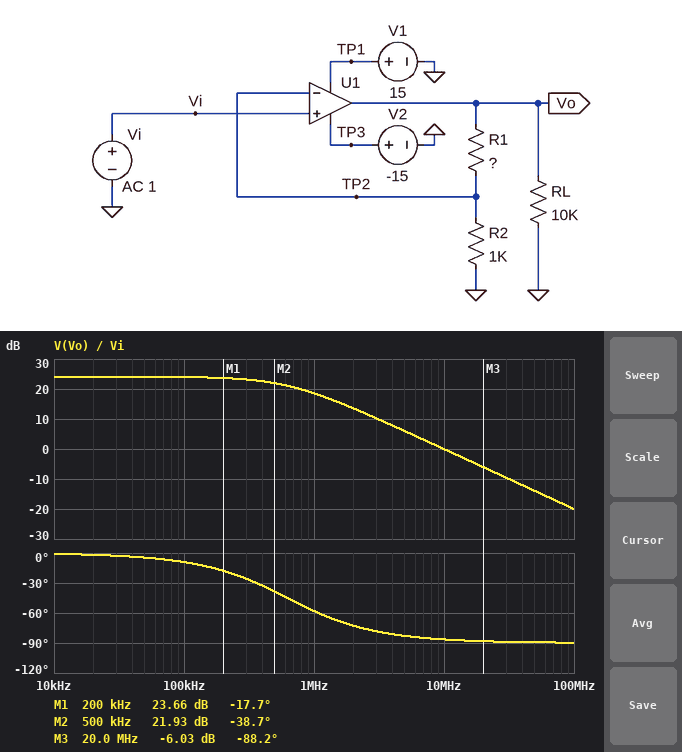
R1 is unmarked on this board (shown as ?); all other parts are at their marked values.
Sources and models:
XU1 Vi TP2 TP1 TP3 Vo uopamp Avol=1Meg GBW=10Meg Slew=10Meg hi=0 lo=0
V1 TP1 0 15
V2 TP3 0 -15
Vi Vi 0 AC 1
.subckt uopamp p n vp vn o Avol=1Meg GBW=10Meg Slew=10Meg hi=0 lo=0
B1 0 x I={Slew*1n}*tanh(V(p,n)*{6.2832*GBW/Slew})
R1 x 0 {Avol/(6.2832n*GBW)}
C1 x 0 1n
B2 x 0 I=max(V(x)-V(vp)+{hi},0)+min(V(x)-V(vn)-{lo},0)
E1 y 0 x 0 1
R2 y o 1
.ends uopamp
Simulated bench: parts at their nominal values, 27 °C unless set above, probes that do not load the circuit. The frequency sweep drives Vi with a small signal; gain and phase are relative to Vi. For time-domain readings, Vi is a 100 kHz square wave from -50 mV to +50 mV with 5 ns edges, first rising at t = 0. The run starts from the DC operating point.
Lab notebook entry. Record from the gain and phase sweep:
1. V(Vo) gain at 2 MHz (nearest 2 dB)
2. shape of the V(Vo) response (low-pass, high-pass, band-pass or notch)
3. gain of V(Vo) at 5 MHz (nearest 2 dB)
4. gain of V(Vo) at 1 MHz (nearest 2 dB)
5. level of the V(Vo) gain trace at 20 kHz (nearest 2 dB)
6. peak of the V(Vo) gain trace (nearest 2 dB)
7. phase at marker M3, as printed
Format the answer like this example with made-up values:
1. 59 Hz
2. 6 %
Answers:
1. 14 dB
2. low-pass
3. 6 dB
4. 18 dB
5. 24 dB
6. 24 dB
7. -88.2 deg
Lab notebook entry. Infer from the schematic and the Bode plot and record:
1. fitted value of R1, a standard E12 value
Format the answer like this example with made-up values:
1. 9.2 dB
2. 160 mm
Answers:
1. 15 kΩ
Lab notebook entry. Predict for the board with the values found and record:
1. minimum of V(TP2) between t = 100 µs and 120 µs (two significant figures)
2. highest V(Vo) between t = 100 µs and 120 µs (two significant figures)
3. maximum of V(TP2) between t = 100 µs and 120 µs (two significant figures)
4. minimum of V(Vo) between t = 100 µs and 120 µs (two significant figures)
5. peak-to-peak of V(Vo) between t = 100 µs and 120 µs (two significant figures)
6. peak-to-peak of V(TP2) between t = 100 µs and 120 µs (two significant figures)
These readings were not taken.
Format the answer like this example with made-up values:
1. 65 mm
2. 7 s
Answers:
1. -50 mV
2. 800 mV
3. 50 mV
4. -800 mV
5. 1.6 V
6. 100 mV
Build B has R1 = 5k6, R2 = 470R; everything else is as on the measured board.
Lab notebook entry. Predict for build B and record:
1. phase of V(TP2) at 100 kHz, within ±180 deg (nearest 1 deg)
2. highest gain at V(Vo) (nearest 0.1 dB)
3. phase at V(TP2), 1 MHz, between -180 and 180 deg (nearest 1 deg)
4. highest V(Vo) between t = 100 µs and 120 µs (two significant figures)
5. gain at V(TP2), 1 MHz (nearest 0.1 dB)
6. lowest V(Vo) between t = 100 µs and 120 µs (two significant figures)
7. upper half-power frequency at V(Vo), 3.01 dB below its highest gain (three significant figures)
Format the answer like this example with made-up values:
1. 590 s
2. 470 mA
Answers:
1. -7 deg
2. 22.2 dB
3. -52 deg
4. 650 mV
5. -4.3 dB
6. -650 mV
7. 774 kHz
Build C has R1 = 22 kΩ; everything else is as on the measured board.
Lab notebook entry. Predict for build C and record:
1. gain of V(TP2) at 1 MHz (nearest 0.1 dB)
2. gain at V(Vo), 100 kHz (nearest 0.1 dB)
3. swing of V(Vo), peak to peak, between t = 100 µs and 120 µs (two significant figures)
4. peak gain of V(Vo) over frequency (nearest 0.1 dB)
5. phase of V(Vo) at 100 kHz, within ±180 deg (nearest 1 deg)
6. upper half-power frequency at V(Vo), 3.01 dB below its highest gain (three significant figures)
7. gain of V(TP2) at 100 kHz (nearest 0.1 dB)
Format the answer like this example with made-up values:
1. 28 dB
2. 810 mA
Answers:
1. -8.0 dB
2. 27.0 dB
3. 2.3 V
4. 27.2 dB
5. -13 deg
6. 435 kHz
7. -0.2 dB
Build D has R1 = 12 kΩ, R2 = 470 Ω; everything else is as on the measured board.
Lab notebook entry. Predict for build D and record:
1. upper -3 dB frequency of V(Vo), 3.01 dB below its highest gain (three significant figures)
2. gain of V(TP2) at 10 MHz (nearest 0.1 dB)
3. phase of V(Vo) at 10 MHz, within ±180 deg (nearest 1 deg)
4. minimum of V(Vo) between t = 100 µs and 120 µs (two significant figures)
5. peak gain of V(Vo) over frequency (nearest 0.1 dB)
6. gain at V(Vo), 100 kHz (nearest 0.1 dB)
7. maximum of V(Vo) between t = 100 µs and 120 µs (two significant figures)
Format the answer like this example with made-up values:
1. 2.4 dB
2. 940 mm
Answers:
1. 377 kHz
2. -28.5 dB
3. -88 deg
4. -1.3 V
5. 28.5 dB
6. 28.2 dB
7. 1.3 V
